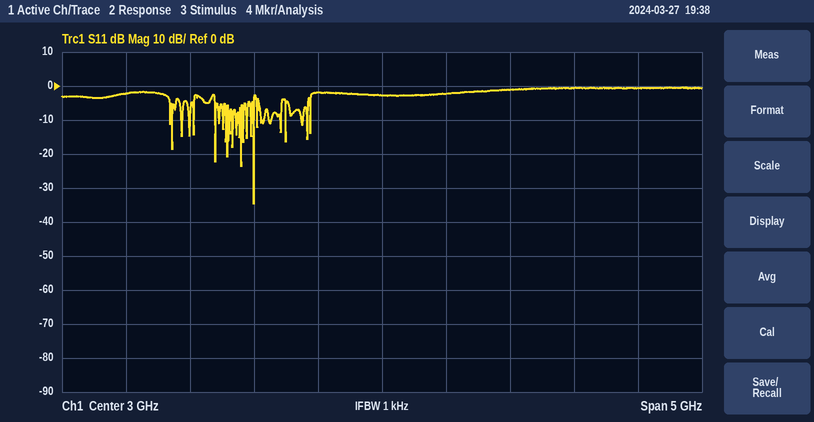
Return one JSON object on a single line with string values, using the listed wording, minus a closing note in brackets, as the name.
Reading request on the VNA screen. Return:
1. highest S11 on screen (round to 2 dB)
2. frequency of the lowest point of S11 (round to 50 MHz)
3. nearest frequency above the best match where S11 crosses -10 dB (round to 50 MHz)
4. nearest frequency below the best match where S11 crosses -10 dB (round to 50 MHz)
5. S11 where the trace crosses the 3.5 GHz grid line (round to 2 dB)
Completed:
{"highest S11 on screen": "0 dB", "frequency of the lowest point of S11": "2.00 GHz", "nearest frequency above the best match where S11 crosses -10 dB": "2.00 GHz", "nearest frequency below the best match where S11 crosses -10 dB": "2.00 GHz", "S11 where the trace crosses the 3.5 GHz grid line": "-2 dB"}
